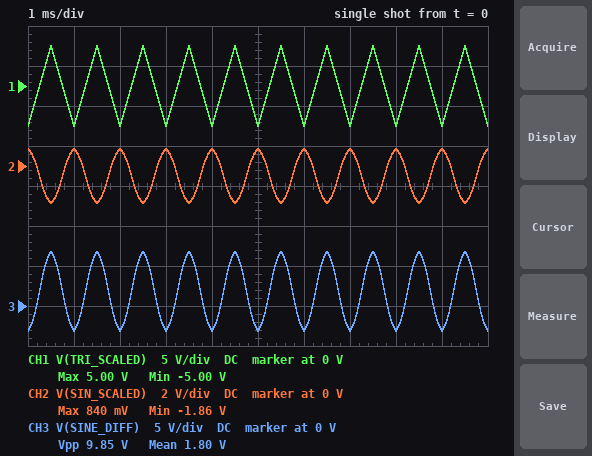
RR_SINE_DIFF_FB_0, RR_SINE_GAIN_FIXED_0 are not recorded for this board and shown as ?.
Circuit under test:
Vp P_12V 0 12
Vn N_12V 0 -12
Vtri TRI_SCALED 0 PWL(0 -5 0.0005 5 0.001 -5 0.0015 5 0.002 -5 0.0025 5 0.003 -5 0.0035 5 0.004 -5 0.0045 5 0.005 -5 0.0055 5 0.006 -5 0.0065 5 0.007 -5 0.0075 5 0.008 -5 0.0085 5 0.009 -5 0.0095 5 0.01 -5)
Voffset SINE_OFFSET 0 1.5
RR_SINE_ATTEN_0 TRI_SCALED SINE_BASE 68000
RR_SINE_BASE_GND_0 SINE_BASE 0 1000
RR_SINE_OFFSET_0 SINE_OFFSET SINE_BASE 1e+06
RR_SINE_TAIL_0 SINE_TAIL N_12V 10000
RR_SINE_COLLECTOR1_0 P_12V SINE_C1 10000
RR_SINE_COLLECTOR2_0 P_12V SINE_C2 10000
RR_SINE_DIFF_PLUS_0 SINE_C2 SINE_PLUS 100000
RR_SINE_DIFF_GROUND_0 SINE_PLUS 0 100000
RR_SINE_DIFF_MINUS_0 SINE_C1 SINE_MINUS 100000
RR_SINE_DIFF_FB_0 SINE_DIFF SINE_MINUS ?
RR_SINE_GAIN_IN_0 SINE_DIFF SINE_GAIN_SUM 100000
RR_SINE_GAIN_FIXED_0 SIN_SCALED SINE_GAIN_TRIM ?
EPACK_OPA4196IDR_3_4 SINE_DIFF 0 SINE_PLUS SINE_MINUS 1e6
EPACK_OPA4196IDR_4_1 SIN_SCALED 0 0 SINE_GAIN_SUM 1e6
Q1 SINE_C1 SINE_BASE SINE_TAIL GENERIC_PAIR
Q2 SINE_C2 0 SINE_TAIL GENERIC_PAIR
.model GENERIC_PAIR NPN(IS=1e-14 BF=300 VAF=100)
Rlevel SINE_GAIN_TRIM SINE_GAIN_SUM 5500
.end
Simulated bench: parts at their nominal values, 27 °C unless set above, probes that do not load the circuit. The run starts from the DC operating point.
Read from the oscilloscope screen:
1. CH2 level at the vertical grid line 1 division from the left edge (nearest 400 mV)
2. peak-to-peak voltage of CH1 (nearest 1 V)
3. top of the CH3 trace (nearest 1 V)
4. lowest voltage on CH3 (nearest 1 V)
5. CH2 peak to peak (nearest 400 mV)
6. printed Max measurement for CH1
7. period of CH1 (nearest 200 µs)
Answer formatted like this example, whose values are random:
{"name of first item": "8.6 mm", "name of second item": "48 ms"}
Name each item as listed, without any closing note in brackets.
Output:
{"CH2 level at the vertical grid line 1 division from the left edge": "800 mV", "peak-to-peak voltage of CH1": "10 V", "top of the CH3 trace": "7 V", "lowest voltage on CH3": "-3 V", "CH2 peak to peak": "2.8 V", "printed Max measurement for CH1": "5.00 V", "period of CH1": "1.0 ms"}
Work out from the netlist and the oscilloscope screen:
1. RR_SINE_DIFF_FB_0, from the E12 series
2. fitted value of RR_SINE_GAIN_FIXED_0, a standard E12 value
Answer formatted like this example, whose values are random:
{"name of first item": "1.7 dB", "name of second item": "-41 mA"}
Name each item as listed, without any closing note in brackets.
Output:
{"RR_SINE_DIFF_FB_0, from the E12 series": "39 kΩ", "fitted value of RR_SINE_GAIN_FIXED_0, a standard E12 value": "22 kΩ"}
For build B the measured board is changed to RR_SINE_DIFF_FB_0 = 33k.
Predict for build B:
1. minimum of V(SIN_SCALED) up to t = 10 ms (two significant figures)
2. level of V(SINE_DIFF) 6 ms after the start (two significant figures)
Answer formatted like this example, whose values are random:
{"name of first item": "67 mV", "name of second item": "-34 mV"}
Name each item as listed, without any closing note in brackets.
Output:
{"minimum of V(SIN_SCALED) up to t = 10 ms": "-1.8 V", "level of V(SINE_DIFF) 6 ms after the start": "-2.5 V"}
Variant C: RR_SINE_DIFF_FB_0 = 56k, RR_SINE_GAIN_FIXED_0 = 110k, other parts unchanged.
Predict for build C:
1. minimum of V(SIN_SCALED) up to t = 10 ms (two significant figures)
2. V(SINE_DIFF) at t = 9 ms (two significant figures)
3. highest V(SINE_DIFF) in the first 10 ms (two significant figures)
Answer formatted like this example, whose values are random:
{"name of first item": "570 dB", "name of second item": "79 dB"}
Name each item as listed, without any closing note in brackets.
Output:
{"minimum of V(SIN_SCALED) up to t = 10 ms": "-8.5 V", "V(SINE_DIFF) at t = 9 ms": "-4.7 V", "highest V(SINE_DIFF) in the first 10 ms": "7.4 V"}
